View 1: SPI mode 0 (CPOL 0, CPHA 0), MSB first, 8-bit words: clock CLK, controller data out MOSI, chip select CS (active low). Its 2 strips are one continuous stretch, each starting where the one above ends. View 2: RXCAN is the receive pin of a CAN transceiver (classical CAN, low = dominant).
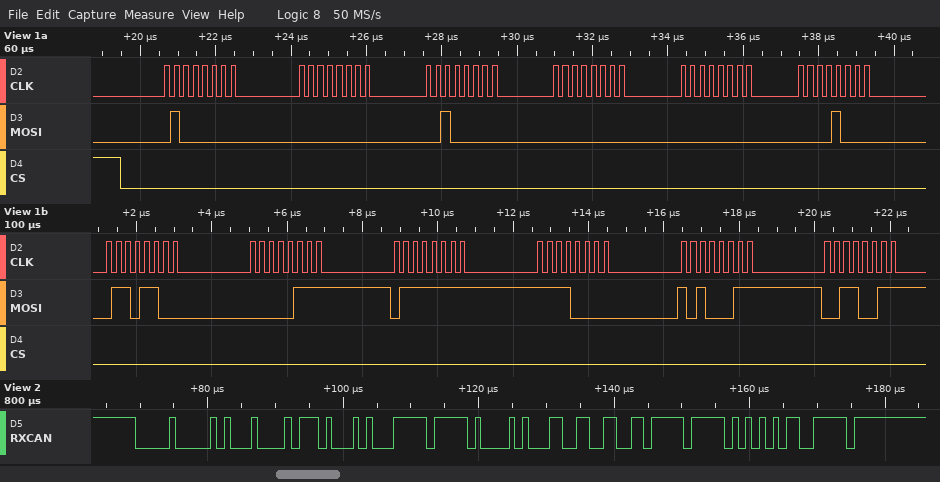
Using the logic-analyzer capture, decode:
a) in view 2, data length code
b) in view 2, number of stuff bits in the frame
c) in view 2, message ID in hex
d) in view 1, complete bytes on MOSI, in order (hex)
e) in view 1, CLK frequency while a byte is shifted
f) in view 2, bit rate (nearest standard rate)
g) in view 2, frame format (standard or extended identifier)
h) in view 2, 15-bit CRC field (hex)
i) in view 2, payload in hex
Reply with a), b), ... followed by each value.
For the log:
a) 8
b) 6
c) 0x001
d) 40 00 20 00 00 08 6C 07 7F F0 A3 33
e) 4 MHz
f) 1000 kbit/s
g) standard
h) 0x2ACF
i) 5D 14 7F F0 A3 33 37 FF
